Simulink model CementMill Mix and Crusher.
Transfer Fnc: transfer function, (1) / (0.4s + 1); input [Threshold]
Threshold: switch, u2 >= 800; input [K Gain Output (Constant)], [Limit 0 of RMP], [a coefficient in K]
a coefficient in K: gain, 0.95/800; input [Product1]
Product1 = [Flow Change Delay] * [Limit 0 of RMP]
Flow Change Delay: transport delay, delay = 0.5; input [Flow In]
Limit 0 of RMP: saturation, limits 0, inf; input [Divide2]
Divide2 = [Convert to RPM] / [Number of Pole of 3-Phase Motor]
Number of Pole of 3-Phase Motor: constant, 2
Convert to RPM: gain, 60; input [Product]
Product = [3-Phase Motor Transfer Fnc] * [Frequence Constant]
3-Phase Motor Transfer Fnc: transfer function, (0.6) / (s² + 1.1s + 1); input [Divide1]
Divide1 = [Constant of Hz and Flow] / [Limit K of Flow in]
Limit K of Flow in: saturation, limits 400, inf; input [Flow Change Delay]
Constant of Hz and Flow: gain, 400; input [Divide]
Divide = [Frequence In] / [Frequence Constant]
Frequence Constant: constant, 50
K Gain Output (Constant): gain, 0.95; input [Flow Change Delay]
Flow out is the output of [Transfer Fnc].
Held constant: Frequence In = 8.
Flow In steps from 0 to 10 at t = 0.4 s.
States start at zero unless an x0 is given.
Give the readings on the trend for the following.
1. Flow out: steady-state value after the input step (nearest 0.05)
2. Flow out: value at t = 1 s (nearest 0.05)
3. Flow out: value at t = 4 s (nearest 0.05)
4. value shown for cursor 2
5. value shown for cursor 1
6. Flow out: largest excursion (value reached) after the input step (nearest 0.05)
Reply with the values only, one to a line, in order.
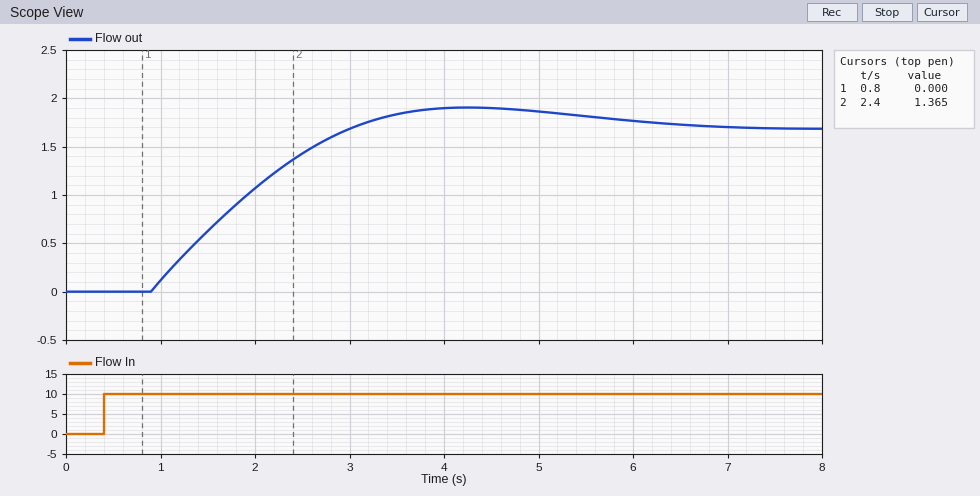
1.70
0.10
1.90
1.365
0.000
1.90
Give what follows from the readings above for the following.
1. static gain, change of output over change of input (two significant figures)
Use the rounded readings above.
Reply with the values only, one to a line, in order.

0.17
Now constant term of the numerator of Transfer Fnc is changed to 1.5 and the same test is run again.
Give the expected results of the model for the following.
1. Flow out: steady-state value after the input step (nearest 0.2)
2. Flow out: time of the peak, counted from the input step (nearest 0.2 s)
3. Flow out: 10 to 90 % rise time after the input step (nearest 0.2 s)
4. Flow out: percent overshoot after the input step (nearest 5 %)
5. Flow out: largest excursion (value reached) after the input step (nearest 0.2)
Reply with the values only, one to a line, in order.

2.6
3.8 s
1.6 s
10 %
2.8
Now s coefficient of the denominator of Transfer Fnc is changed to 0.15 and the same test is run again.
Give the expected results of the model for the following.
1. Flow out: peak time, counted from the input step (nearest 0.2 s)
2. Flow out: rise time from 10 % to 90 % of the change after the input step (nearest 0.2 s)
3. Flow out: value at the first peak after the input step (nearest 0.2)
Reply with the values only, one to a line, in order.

3.6 s
1.4 s
2.0
